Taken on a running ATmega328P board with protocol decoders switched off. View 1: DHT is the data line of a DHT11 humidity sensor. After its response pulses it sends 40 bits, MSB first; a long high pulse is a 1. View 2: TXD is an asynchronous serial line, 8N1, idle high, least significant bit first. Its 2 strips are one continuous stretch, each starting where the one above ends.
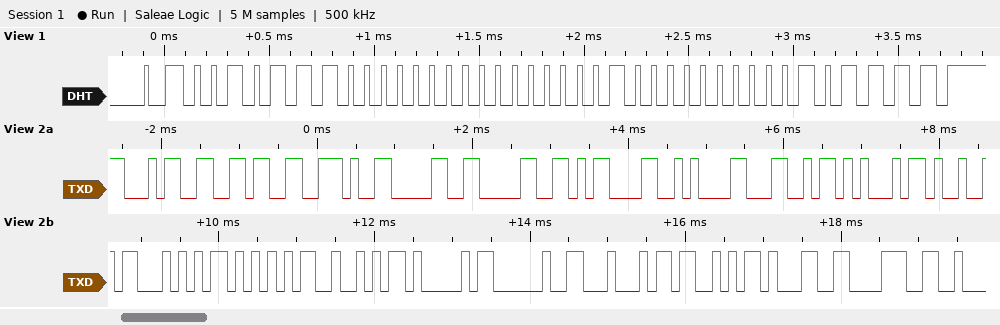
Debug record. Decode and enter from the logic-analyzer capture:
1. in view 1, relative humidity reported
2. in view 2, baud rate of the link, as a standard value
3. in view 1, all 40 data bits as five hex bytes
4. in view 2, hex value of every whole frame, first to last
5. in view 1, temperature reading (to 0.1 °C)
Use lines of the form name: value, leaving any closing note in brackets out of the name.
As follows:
in view 1, relative humidity reported: 46 %
in view 2, baud rate of the link, as a standard value: 9600 baud
in view 1, all 40 data bits as five hex bytes: 2E 00 01 00 2F
in view 2, hex value of every whole frame, first to last: 34 36 2E 30 30 0D 0A 4C 45 49 54 55 52 41 20 44 53 31 38
in view 1, temperature reading: 1.0 °C
